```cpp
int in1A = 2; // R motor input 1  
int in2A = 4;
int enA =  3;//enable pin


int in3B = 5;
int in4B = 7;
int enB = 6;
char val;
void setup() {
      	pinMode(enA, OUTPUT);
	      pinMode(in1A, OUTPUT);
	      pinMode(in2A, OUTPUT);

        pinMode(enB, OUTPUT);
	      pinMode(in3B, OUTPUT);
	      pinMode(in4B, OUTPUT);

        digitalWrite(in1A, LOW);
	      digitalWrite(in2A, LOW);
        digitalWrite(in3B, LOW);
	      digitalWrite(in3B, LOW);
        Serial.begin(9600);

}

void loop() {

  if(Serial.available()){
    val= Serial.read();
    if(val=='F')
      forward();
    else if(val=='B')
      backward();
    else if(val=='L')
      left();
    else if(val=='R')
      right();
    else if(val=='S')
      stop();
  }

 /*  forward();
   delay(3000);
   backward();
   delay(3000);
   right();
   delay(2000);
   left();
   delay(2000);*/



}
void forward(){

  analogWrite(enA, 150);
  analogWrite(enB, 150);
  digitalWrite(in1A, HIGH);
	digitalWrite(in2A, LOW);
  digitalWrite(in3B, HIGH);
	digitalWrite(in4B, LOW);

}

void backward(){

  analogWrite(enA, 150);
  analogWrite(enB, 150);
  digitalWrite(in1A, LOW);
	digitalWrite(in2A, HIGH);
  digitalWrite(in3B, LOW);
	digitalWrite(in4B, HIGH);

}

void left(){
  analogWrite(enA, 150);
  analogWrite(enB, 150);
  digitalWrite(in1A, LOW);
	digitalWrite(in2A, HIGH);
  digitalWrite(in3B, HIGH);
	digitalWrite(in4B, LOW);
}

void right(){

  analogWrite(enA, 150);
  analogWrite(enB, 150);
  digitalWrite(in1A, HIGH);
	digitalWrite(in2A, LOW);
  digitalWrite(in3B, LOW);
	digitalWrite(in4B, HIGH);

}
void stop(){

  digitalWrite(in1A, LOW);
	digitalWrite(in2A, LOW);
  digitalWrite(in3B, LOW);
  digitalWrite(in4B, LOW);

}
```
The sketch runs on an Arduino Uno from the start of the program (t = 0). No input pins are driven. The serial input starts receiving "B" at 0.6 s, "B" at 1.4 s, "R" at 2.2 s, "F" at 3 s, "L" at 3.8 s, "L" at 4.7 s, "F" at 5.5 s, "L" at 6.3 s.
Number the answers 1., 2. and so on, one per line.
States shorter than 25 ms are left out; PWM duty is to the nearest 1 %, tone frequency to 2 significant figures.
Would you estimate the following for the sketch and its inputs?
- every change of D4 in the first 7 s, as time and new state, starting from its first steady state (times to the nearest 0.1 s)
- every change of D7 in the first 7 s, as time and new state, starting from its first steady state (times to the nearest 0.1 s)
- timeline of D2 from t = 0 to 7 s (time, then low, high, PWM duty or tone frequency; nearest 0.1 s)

1. 0 s low; 0.6 s high; 2.2 s low; 3.8 s high; 5.5 s low; 6.3 s high
2. 0 s low; 0.6 s high; 3 s low
3. 0 s low; 2.2 s high; 3.8 s low; 5.5 s high; 6.3 s low
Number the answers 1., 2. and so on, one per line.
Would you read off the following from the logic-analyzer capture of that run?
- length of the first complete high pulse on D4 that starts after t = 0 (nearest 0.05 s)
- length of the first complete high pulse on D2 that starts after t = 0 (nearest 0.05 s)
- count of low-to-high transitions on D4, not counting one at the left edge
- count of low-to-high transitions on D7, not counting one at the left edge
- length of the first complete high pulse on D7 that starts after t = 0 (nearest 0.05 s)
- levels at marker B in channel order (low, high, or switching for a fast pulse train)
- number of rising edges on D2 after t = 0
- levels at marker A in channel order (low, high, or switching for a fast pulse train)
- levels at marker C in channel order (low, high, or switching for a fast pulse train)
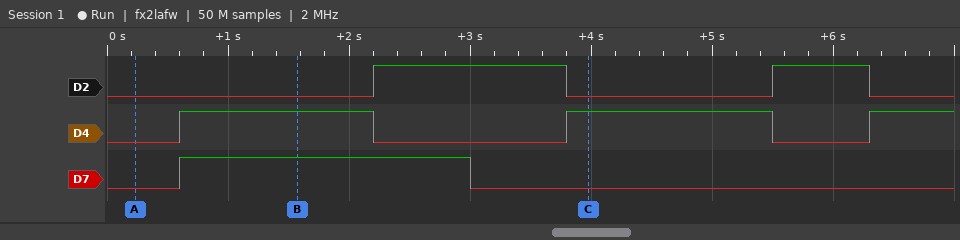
1. 1.60 s
2. 1.60 s
3. 3
4. 1
5. 2.40 s
6. D2 low, D4 high, D7 high
7. 2
8. D2 low, D4 low, D7 low
9. D2 low, D4 high, D7 low
